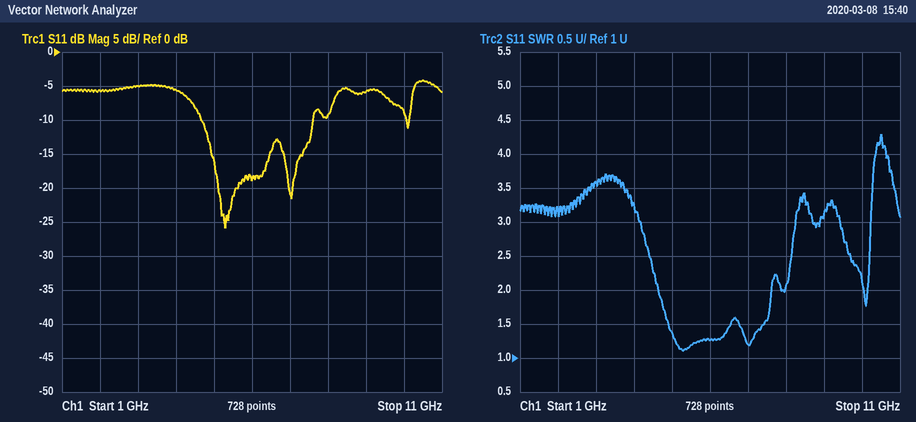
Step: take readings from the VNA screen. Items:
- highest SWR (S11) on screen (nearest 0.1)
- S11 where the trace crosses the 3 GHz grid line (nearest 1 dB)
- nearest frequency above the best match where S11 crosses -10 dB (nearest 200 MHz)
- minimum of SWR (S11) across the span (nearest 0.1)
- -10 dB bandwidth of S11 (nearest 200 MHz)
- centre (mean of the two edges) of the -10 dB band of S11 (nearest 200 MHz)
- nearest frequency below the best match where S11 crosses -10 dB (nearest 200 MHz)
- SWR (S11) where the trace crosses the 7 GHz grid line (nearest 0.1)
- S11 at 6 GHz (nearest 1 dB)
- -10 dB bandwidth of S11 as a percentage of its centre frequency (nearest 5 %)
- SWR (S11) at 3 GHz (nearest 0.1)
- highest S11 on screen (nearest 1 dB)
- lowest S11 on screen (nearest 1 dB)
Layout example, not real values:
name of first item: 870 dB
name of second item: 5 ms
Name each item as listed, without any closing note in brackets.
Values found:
highest SWR (S11) on screen: 4.3
S11 where the trace crosses the 3 GHz grid line: -5 dB
nearest frequency above the best match where S11 crosses -10 dB: 7.6 GHz
minimum of SWR (S11) across the span: 1.1
-10 dB bandwidth of S11: 3.0 GHz
centre (mean of the two edges) of the -10 dB band of S11: 6.2 GHz
nearest frequency below the best match where S11 crosses -10 dB: 4.6 GHz
SWR (S11) where the trace crosses the 7 GHz grid line: 1.2
S11 at 6 GHz: -19 dB
-10 dB bandwidth of S11 as a percentage of its centre frequency: 50 %
SWR (S11) at 3 GHz: 3.6
highest S11 on screen: -4 dB
lowest S11 on screen: -26 dB
